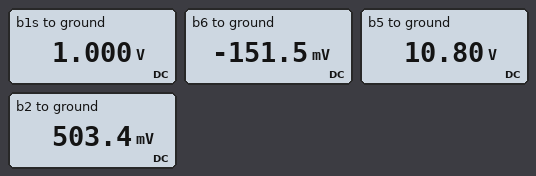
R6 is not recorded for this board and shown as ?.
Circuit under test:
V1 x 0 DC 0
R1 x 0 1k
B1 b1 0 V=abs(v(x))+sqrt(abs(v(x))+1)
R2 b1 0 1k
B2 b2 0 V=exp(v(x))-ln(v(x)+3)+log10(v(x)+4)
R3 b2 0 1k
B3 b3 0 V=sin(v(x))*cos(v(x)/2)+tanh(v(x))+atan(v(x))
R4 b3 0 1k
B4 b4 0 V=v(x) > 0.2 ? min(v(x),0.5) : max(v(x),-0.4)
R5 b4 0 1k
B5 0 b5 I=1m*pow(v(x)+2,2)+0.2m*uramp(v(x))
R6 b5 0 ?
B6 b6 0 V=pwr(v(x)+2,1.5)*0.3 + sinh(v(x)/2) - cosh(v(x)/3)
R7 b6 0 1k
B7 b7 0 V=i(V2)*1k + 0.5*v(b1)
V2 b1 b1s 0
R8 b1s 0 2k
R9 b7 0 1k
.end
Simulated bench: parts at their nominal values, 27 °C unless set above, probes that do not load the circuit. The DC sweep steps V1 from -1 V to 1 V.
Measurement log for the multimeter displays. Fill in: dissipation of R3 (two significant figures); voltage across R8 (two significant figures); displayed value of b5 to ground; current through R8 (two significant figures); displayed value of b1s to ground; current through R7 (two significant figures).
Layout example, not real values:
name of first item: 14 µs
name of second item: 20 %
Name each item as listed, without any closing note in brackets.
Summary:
dissipation of R3: 250 µW
voltage across R8: 1.0 V
displayed value of b5 to ground: 10.80 V
current through R8: 500 µA
displayed value of b1s to ground: 1.000 V
current through R7: 150 µA
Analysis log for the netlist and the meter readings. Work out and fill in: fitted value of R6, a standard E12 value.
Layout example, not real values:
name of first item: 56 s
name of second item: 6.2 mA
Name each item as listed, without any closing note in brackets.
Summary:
fitted value of R6, a standard E12 value: 2.7 kΩ
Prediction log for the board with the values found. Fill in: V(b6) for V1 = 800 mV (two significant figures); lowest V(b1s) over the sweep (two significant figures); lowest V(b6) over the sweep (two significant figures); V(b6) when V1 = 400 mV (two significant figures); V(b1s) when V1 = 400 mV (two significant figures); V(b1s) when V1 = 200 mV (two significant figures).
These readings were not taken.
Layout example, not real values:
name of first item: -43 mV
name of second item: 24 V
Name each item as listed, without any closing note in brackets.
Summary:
V(b6) for V1 = 800 mV: 780 mV
lowest V(b1s) over the sweep: 1.0 V
lowest V(b6) over the sweep: -1.3 V
V(b6) when V1 = 400 mV: 310 mV
V(b1s) when V1 = 400 mV: 1.6 V
V(b1s) when V1 = 200 mV: 1.3 V
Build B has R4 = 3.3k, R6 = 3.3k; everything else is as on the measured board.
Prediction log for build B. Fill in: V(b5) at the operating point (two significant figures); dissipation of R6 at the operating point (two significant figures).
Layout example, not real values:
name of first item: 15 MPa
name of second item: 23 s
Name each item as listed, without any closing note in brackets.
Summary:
V(b5) at the operating point: 13 V
dissipation of R6 at the operating point: 53 mW
